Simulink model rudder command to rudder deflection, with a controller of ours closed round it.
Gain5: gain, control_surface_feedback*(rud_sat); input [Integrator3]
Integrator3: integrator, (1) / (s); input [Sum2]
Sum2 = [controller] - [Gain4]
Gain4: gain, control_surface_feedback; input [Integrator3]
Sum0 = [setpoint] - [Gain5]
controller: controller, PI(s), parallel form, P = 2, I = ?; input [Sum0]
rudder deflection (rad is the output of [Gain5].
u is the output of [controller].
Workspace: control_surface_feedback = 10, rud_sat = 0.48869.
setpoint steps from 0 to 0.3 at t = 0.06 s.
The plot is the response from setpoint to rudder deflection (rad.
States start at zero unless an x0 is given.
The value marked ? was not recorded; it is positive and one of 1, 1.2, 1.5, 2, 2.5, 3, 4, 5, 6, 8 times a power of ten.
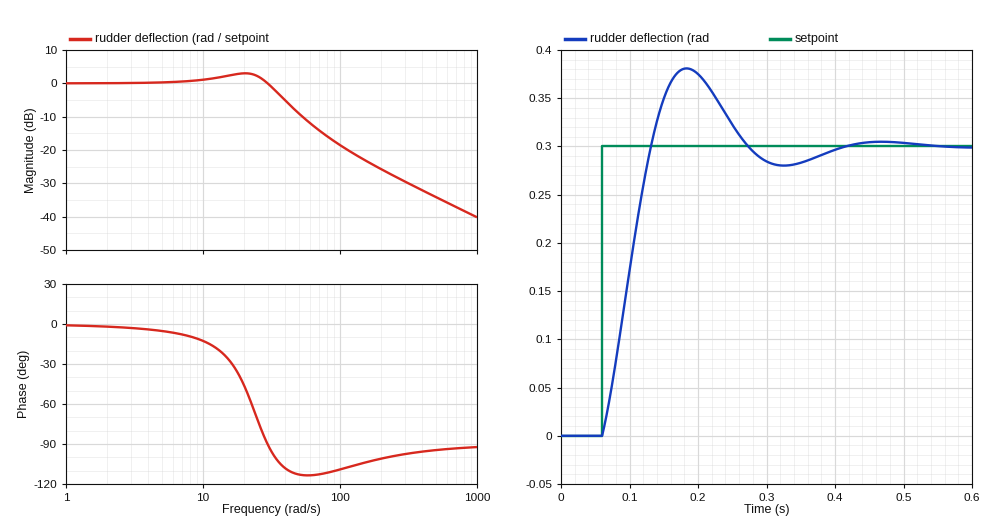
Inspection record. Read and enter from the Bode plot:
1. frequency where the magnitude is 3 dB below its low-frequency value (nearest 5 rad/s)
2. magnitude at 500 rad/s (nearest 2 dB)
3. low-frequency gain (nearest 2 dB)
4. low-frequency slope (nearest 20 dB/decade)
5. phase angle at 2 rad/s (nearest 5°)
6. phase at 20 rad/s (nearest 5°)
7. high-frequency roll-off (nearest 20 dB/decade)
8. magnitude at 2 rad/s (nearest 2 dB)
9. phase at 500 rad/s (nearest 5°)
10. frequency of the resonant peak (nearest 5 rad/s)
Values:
35 rad/s
-34 dB
0 dB
0 dB/decade
0°
-45°
-20 dB/decade
0 dB
-95°
20 rad/s
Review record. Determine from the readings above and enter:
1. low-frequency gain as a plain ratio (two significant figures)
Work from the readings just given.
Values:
1.0
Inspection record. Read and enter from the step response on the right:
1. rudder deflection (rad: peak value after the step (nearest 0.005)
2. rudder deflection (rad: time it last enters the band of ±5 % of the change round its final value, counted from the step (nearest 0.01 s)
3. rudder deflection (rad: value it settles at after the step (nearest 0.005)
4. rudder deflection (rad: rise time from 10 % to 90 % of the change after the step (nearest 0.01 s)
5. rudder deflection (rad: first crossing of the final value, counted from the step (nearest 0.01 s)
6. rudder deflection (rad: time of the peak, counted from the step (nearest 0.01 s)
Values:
0.380
0.30 s
0.300
0.05 s
0.07 s
0.12 s
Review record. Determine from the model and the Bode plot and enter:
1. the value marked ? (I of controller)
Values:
120
